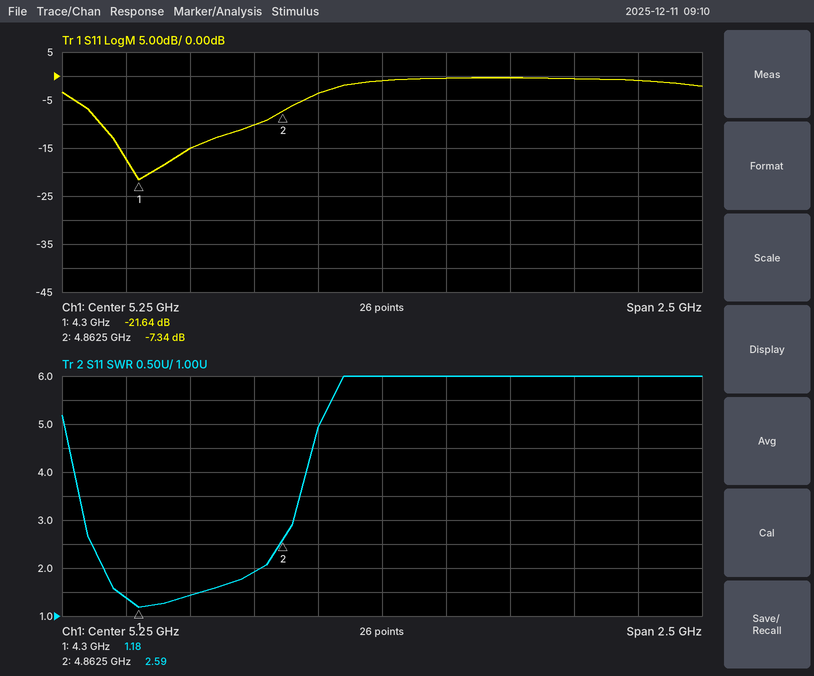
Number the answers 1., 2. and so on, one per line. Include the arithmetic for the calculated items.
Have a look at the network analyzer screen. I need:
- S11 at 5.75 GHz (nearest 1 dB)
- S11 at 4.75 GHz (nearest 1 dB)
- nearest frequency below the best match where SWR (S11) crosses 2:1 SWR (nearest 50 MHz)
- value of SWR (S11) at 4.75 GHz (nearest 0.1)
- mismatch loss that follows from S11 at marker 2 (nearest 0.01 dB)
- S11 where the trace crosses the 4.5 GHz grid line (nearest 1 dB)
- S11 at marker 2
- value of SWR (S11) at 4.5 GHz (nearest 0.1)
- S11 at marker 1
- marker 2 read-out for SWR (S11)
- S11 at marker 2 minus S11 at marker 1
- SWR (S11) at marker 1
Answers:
1. 0 dB
2. -10 dB
3. 4.15 GHz
4. 1.9
5. −10 log10(1 − 10^(-7.34/10)) ≈ 0.89 dB
6. -15 dB
7. -7.34 dB
8. 1.4
9. -21.64 dB
10. 2.59
11. -7.34 − (-21.64) = 14.30 dB
12. 1.18
